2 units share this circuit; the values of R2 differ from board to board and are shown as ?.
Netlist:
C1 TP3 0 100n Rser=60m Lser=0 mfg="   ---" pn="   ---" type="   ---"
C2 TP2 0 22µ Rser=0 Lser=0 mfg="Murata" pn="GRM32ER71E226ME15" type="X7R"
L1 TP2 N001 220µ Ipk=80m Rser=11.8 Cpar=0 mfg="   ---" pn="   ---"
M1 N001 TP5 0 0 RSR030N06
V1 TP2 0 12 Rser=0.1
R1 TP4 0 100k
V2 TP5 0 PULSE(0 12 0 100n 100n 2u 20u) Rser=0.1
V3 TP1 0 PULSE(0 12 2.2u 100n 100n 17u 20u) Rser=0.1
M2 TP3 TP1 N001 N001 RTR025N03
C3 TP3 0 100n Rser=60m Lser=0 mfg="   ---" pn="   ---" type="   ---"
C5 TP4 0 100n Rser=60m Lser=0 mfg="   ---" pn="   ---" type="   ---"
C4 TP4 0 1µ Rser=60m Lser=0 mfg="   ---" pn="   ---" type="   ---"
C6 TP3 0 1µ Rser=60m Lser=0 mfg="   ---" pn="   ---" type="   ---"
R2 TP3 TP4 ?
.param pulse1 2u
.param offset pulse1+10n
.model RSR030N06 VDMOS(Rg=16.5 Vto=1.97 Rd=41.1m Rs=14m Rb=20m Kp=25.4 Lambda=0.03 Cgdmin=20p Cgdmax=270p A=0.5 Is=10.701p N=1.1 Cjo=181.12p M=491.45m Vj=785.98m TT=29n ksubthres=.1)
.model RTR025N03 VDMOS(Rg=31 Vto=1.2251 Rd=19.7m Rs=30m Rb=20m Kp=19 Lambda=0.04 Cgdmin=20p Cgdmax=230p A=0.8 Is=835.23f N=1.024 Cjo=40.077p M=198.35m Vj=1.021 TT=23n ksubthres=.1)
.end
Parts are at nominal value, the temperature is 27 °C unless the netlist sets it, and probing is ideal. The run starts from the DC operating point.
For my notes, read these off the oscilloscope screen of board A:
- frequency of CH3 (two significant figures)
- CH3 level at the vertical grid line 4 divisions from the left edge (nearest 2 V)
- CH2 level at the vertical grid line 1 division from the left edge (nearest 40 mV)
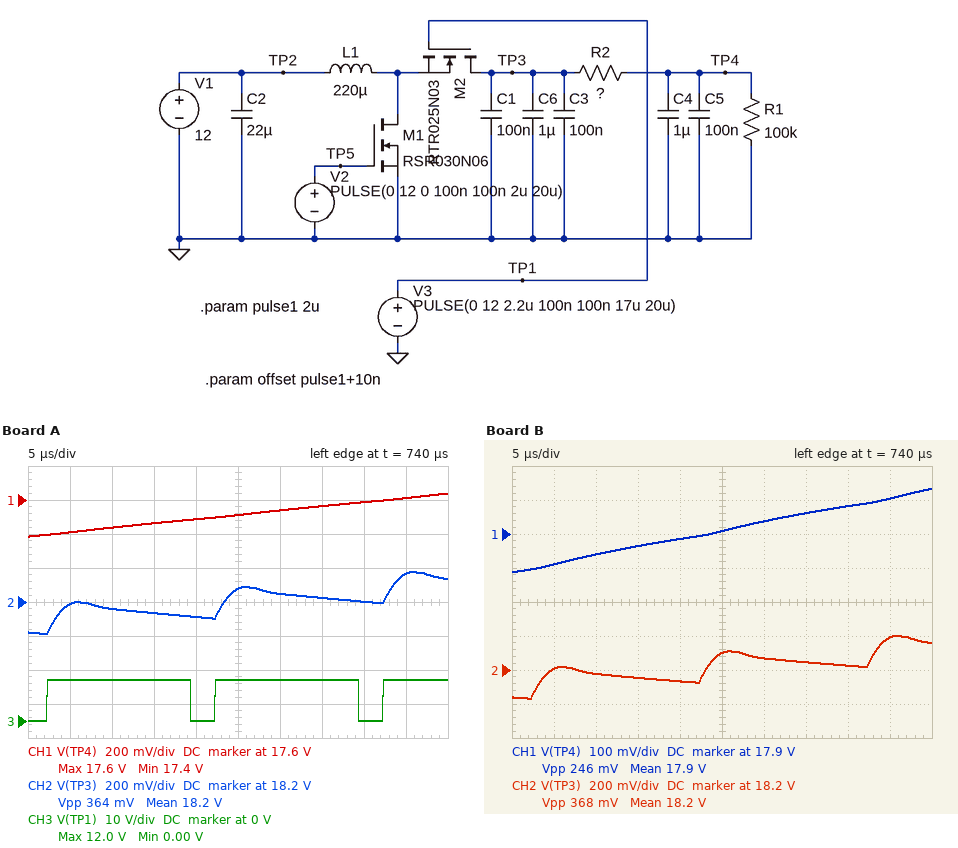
50 kHz
0 V
18.20 V
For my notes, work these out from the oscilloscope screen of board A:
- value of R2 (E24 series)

120 Ω
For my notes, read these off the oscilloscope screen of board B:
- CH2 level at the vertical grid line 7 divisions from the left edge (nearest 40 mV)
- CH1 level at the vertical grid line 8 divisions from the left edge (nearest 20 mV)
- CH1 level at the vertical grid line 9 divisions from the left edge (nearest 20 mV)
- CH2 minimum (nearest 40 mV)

18.24 V
17.98 V
18.00 V
18.04 V
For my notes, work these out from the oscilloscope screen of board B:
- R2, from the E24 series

56 Ω
